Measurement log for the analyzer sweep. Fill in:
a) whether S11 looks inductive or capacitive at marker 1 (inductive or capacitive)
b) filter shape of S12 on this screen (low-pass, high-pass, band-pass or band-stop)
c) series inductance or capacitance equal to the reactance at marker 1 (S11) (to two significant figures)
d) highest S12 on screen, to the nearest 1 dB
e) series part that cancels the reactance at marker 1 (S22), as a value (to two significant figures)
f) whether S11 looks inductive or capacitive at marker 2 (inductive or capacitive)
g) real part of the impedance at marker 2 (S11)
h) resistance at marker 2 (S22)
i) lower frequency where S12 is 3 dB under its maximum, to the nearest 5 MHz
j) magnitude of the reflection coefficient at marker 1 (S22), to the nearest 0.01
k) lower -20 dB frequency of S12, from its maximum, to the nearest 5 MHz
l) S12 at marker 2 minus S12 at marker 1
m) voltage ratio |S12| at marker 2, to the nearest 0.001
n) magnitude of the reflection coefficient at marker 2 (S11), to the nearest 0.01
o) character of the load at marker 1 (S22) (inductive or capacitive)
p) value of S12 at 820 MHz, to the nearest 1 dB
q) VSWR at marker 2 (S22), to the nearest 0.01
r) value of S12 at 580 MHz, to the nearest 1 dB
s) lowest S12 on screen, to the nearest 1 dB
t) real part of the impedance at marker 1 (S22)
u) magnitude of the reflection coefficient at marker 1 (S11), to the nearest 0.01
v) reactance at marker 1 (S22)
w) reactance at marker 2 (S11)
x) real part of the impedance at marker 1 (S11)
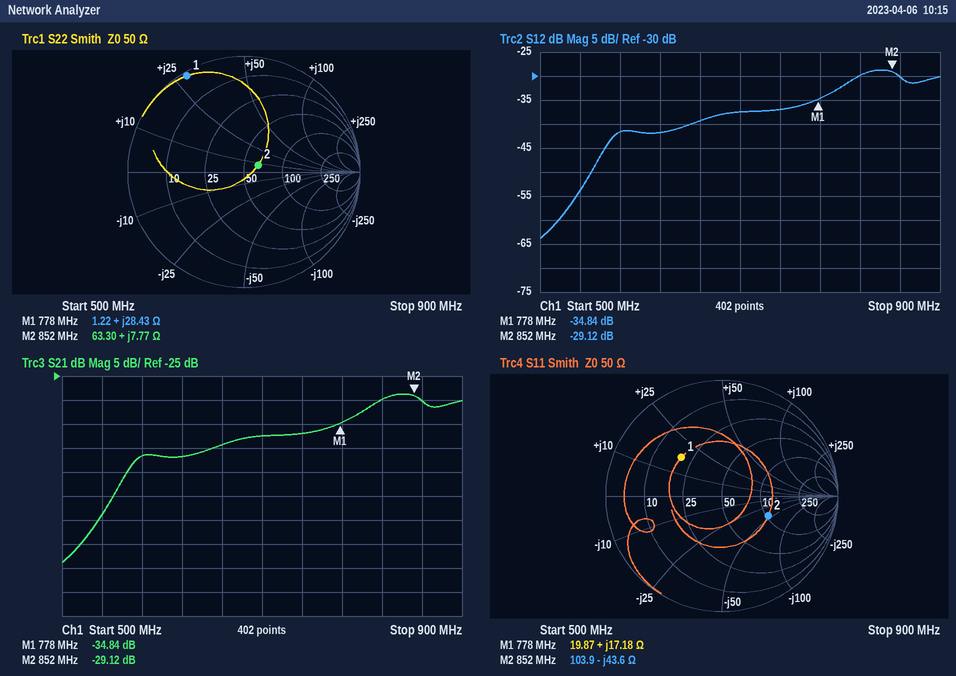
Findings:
inductive
high-pass
3.5 nH
-29 dB
7.2 pF
capacitive
103.9 Ω
63.30 Ω
805 MHz
0.96
555 MHz
5.72 dB
0.035
0.43
inductive
-30 dB
1.31
-42 dB
-64 dB
1.22 Ω
0.48
+28.43 Ω
-43.6 Ω
19.87 Ω
